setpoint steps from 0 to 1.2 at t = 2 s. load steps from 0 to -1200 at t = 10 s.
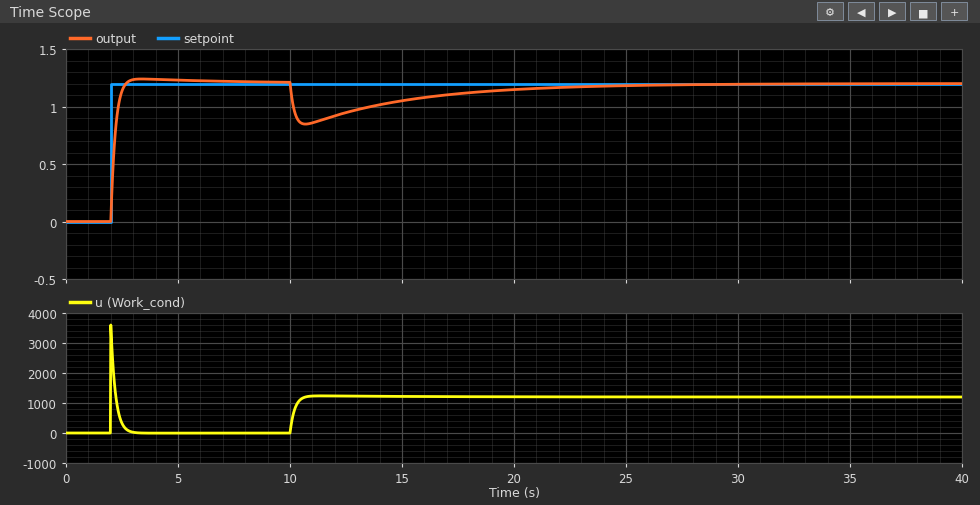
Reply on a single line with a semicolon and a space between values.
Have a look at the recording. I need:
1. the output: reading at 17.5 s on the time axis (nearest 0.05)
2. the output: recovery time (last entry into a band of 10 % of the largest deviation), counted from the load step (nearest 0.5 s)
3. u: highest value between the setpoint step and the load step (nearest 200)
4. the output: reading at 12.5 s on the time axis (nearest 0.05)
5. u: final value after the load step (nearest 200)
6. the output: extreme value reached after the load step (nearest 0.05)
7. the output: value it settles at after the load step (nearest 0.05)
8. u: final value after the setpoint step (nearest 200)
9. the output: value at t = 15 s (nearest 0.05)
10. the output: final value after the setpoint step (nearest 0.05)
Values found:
1.10; 12.0 s; 3600; 0.95; 1200; 0.85; 1.20; 0; 1.05; 1.20
